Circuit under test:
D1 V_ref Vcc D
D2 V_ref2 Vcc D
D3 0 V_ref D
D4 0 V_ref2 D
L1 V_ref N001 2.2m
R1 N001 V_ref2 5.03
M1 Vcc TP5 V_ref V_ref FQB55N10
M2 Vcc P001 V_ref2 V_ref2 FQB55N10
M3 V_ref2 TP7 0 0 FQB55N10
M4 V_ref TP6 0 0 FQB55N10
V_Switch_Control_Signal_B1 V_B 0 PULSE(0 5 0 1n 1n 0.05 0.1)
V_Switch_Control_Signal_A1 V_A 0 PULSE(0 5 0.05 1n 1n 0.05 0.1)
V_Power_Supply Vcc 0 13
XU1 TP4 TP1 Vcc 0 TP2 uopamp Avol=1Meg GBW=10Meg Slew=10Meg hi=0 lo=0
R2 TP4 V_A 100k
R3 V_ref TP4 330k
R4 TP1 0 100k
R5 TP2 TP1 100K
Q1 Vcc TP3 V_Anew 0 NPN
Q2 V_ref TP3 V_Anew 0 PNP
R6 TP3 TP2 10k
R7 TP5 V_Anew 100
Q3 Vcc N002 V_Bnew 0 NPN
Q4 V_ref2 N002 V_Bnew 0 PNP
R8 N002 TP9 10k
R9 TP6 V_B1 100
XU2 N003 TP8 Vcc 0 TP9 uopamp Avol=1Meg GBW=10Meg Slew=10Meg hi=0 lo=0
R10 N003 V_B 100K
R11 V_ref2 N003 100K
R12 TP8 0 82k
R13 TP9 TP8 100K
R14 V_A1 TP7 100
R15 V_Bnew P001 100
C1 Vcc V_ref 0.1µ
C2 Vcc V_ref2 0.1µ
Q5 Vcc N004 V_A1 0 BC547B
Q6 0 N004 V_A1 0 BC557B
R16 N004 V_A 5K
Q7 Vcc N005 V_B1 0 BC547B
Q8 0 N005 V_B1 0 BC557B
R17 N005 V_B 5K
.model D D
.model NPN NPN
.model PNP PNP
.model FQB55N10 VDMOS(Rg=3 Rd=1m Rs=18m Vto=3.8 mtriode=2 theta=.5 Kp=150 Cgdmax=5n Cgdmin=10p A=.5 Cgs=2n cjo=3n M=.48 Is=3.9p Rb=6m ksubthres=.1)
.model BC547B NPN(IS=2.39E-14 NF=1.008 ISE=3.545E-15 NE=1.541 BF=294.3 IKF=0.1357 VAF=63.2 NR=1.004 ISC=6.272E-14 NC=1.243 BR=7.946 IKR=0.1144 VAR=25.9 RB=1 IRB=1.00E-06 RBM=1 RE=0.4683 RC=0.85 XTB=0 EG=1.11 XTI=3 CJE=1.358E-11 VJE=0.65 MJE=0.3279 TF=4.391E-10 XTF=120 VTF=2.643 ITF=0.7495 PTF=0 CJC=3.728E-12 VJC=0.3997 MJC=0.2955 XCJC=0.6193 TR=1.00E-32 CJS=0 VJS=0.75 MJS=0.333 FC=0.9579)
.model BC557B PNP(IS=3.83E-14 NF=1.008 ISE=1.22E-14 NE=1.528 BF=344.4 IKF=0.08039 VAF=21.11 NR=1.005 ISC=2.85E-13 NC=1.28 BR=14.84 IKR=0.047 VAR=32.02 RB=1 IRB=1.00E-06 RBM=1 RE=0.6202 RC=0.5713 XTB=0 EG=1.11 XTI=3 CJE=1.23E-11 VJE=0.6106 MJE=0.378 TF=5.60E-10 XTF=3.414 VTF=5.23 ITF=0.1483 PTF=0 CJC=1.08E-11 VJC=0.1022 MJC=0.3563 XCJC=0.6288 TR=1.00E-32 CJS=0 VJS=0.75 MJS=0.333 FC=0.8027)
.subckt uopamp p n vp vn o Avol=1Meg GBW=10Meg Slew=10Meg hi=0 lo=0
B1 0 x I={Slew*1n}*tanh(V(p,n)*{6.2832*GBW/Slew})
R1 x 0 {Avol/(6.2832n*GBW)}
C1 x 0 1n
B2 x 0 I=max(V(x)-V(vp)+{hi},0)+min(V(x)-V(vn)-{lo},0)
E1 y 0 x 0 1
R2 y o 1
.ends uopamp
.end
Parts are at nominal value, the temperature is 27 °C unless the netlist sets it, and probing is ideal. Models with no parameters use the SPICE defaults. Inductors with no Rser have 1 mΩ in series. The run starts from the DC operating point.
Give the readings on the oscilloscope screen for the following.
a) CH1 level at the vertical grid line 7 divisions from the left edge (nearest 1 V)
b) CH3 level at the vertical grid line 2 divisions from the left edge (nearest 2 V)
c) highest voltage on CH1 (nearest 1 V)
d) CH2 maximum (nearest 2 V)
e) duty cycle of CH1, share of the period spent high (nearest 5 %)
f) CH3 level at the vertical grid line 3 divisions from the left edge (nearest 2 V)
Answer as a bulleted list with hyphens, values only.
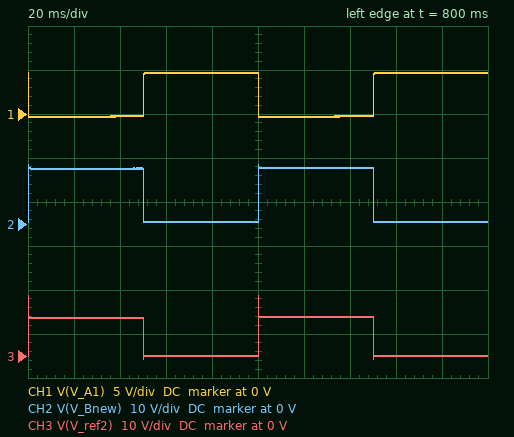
- 0 V
- 8 V
- 5 V
- 14 V
- 50 %
- 0 V
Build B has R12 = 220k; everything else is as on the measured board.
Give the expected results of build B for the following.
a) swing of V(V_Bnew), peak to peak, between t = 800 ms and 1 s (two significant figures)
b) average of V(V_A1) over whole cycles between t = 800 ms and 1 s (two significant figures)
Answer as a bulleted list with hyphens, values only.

- 12 V
- 2.3 V
